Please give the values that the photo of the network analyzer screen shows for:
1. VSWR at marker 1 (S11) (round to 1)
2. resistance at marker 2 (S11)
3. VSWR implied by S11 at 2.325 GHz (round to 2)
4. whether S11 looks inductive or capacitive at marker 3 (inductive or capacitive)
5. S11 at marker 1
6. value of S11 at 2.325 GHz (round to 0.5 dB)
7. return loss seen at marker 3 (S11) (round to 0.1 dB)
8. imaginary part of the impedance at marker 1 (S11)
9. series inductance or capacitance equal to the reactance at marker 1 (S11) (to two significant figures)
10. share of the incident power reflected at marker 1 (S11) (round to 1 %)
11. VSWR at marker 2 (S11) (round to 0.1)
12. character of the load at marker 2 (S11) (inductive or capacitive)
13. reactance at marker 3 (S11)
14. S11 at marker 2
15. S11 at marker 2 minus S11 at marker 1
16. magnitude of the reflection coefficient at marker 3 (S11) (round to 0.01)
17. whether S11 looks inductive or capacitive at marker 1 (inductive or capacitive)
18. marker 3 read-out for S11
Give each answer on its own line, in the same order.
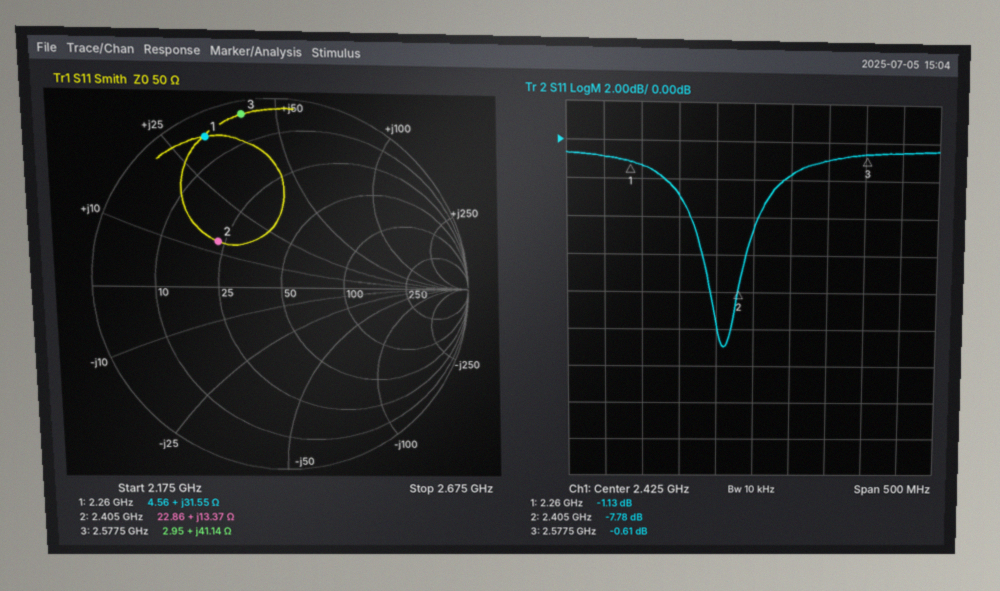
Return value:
15
22.86 Ω
6
inductive
-1.13 dB
-3.0 dB
0.6 dB
+31.55 Ω
2.2 nH
77 %
2.4
inductive
+41.14 Ω
-7.78 dB
-6.65 dB
0.93
inductive
-0.61 dB
